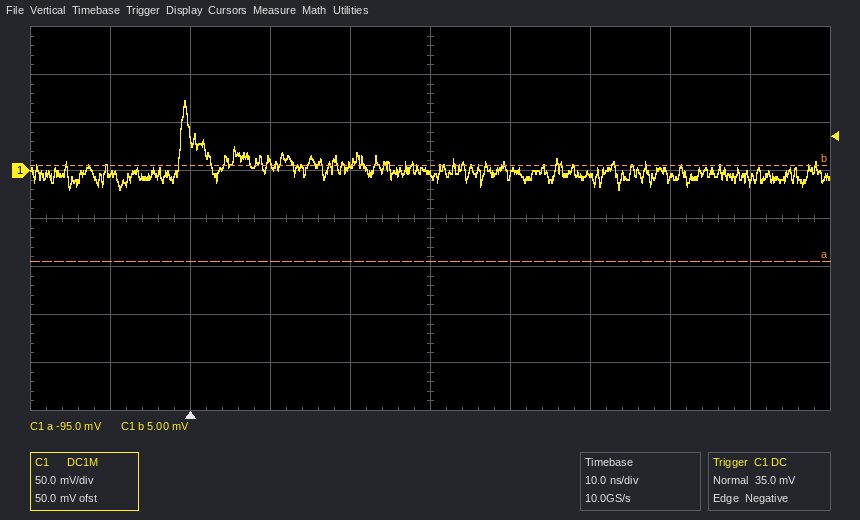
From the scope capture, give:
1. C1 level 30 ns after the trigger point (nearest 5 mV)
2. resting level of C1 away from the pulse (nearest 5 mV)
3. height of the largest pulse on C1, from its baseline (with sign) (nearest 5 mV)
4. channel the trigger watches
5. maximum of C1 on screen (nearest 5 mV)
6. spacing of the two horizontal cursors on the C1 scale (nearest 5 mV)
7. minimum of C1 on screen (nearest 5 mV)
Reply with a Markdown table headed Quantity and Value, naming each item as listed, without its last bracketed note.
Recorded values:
| Quantity | Value |
|---|---|
| C1 level 30 ns after the trigger point | -5 mV |
| resting level of C1 away from the pulse | 0 mV |
| height of the largest pulse on C1, from its baseline (with sign) | +75 mV |
| channel the trigger watches | C1 |
| maximum of C1 on screen | 75 mV |
| spacing of the two horizontal cursors on the C1 scale | 100 mV |
| minimum of C1 on screen | -20 mV |
